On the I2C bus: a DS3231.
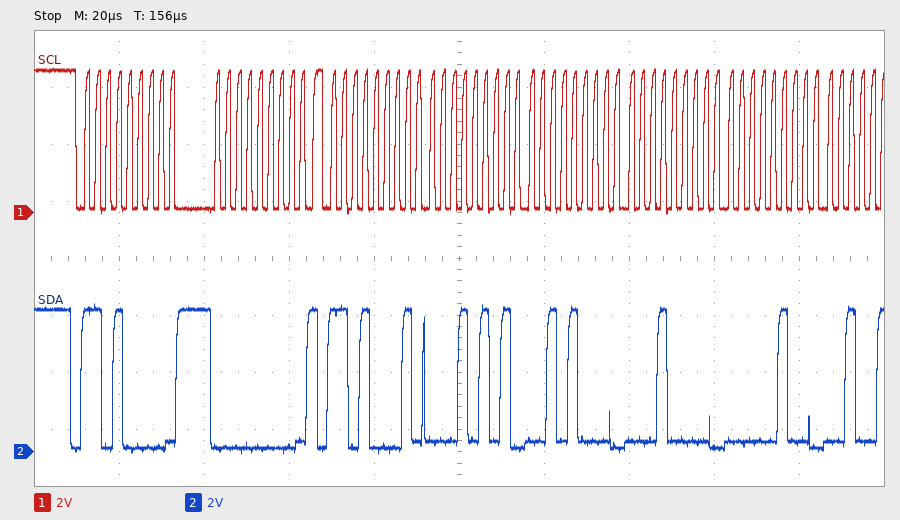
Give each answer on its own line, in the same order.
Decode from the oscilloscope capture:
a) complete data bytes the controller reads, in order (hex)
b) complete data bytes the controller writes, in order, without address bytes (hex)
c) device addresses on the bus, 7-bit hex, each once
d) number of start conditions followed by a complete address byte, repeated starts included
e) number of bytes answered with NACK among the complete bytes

15 28 10 04
00
0x68
2
0
